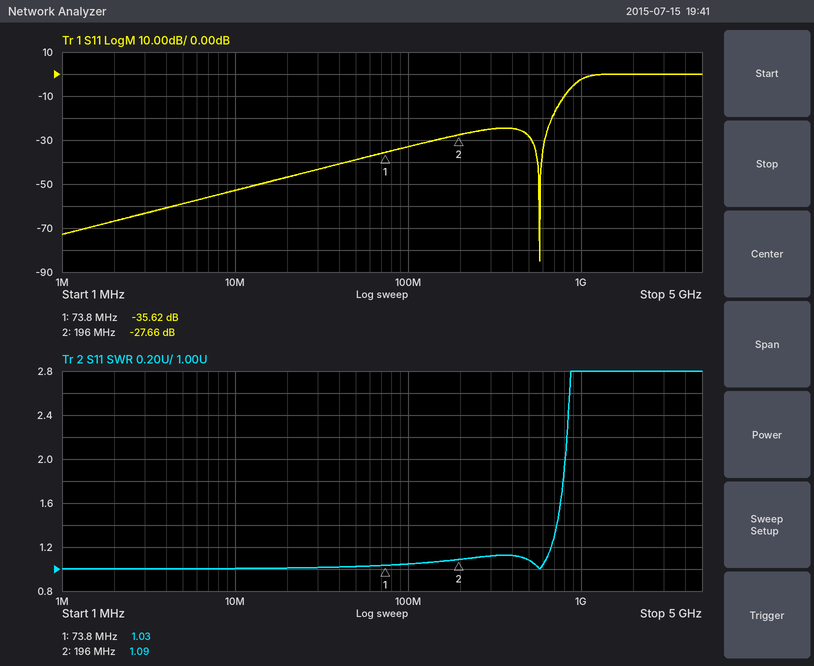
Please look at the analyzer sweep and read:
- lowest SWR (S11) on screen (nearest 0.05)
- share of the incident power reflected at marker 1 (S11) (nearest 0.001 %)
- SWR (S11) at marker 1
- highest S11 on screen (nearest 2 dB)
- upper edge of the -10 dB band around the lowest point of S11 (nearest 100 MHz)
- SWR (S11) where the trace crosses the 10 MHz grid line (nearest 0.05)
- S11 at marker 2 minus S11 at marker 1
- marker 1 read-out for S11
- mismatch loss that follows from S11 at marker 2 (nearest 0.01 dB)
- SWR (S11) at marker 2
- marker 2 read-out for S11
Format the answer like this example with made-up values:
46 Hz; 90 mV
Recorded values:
1.00; 0.027 %; 1.03; 0 dB; 800 MHz; 1.00; 7.96 dB; -35.62 dB; 0.01 dB; 1.09; -27.66 dB
